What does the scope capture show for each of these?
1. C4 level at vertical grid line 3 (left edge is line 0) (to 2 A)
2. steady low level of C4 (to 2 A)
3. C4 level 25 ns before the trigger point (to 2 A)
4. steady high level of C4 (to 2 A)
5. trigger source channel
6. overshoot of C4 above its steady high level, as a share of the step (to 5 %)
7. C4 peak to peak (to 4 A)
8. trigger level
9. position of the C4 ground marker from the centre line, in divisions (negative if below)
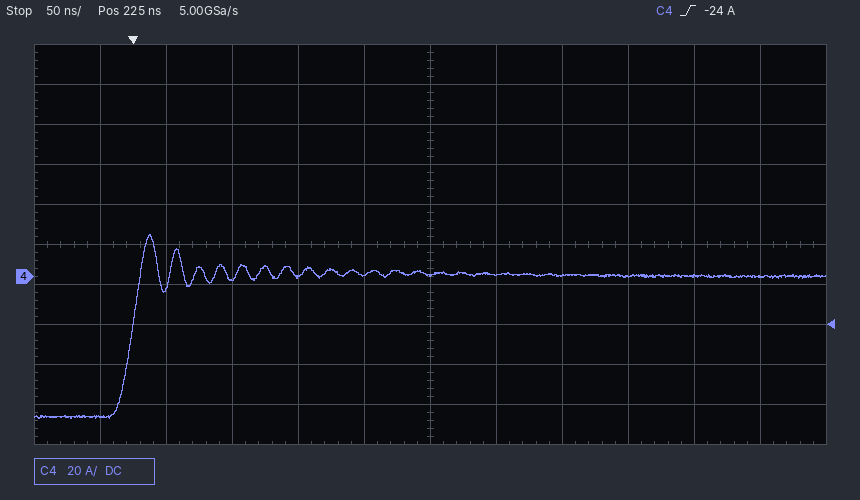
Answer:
-2 A
-70 A
-70 A
0 A
C4
30 %
92 A
-24 A
-0.8 div
